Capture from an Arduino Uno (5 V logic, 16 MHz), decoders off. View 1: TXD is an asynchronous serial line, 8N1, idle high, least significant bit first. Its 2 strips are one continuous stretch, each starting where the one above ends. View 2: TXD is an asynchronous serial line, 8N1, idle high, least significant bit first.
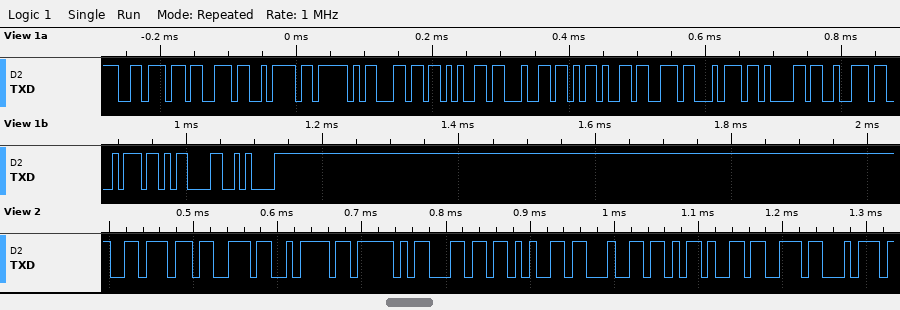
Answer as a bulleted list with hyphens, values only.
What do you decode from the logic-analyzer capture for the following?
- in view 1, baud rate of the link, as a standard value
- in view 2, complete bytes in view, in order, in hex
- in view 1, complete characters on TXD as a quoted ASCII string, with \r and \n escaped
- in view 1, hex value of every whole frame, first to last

- 115200 baud
- 76 73 7A 5F 6C 65 64 2D 73 74
- "vsz_led-start\r\n"
- 76 73 7A 5F 6C 65 64 2D 73 74 61 72 74 0D 0A
